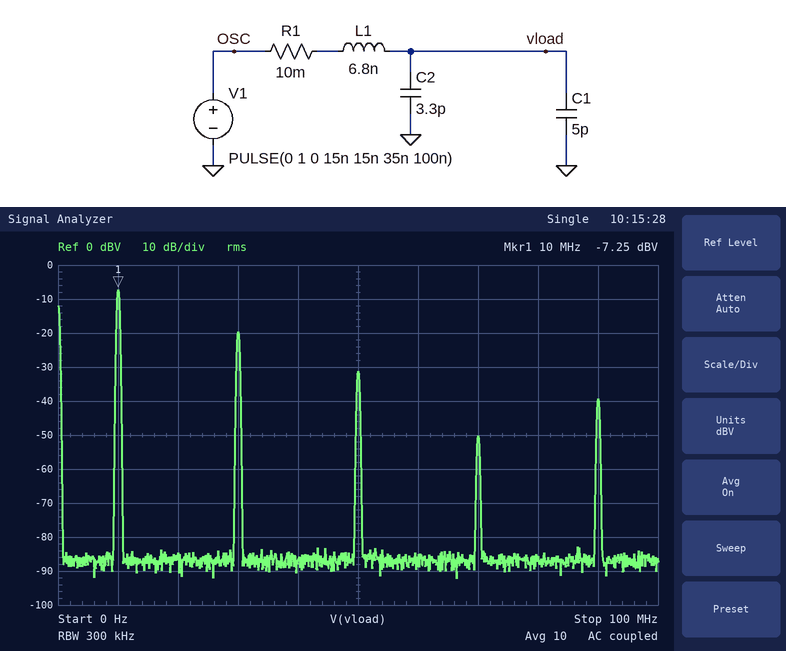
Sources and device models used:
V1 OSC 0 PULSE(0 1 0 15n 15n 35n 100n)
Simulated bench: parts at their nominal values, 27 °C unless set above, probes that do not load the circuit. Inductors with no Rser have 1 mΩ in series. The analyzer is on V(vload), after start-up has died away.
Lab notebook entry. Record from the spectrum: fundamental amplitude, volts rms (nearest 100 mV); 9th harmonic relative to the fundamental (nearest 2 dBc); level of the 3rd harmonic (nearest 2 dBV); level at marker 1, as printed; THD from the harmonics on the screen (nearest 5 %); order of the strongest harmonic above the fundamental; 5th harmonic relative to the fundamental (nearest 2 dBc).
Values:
400 mV
-32 dBc
-20 dBV
-7.25 dBV
25 %
3
-24 dBc
